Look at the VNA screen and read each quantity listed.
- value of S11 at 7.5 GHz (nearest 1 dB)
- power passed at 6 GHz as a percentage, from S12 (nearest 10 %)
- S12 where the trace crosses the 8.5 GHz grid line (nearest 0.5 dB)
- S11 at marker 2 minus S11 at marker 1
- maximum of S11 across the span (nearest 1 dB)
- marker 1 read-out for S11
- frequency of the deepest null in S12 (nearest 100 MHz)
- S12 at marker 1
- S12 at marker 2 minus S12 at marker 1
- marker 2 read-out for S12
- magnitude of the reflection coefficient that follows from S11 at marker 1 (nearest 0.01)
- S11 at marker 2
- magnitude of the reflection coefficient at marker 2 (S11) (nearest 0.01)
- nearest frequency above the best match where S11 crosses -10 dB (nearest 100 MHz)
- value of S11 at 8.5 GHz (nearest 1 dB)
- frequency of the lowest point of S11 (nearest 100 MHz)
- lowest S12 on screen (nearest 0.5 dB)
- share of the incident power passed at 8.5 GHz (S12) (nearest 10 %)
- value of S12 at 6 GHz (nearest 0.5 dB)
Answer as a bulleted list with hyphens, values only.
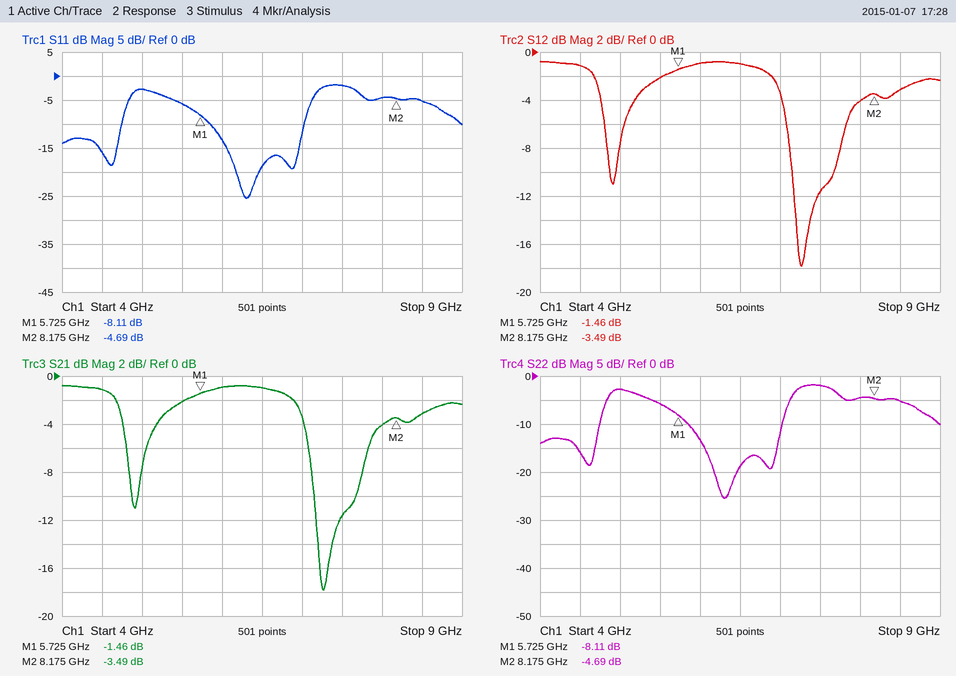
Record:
- -2 dB
- 80 %
- -3.0 dB
- 3.42 dB
- -2 dB
- -8.11 dB
- 7.3 GHz
- -1.46 dB
- -2.03 dB
- -3.49 dB
- 0.39
- -4.69 dB
- 0.58
- 7.0 GHz
- -5 dB
- 6.3 GHz
- -18.0 dB
- 50 %
- -1.0 dB
